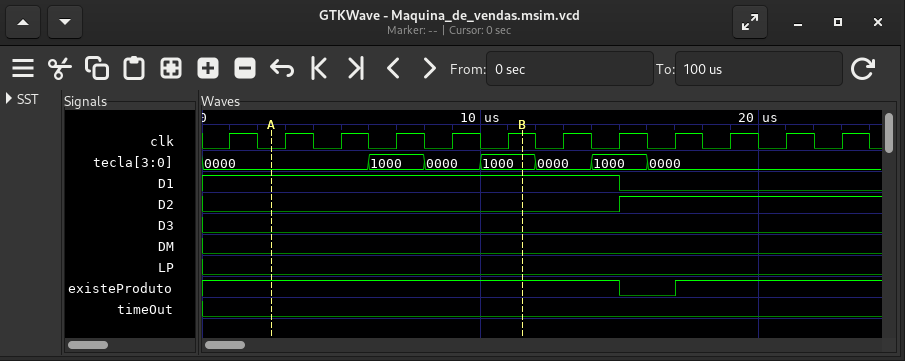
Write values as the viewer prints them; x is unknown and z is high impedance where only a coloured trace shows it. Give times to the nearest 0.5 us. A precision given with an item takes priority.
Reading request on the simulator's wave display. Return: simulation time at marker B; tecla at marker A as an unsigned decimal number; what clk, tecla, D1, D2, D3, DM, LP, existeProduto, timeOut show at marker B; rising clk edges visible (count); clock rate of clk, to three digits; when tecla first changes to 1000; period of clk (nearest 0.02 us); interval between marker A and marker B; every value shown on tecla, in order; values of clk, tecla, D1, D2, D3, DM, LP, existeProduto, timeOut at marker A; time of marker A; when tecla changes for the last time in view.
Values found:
11.5 us
0
clk=1, tecla=1000, D1=1, D2=0, D3=0, DM=0, LP=0, existeProduto=1, timeOut=0
12
500 kHz
6 us
2 us
9 us
0000, 1000, 0000, 1000, 0000, 1000, 0000
clk=0, tecla=0000, D1=1, D2=0, D3=0, DM=0, LP=0, existeProduto=1, timeOut=0
2.5 us
16 us
